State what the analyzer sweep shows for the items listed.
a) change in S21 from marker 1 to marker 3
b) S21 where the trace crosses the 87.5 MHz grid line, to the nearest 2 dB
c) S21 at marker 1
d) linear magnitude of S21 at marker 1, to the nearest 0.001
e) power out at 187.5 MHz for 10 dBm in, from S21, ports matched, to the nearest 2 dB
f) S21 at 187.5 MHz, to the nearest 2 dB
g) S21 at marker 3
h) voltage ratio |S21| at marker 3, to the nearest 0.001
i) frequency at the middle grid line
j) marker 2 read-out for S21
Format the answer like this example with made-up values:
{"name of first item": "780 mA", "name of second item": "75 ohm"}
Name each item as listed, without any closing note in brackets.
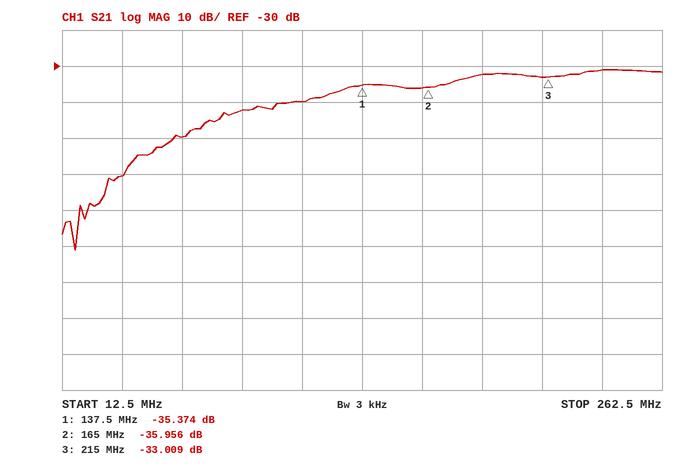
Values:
{"change in S21 from marker 1 to marker 3": "2.365 dB", "S21 where the trace crosses the 87.5 MHz grid line, to the nearest 2 dB": "-42 dB", "S21 at marker 1": "-35.374 dB", "linear magnitude of S21 at marker 1, to the nearest 0.001": "0.017", "power out at 187.5 MHz for 10 dBm in, from S21, ports matched, to the nearest 2 dB": "-22 dBm", "S21 at 187.5 MHz, to the nearest 2 dB": "-32 dB", "S21 at marker 3": "-33.009 dB", "voltage ratio |S21| at marker 3, to the nearest 0.001": "0.022", "frequency at the middle grid line": "137.5 MHz", "marker 2 read-out for S21": "-35.956 dB"}
